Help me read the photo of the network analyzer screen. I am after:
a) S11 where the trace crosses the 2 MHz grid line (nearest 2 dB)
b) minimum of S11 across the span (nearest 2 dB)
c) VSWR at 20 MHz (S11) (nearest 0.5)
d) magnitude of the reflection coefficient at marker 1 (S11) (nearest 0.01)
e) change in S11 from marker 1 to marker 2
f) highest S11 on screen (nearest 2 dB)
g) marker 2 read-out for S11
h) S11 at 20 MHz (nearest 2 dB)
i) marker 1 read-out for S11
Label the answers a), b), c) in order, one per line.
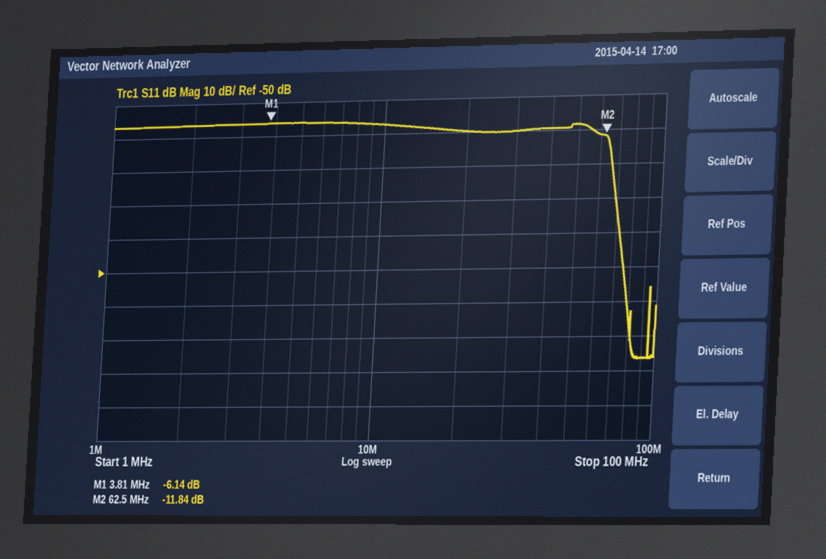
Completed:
a) -6 dB
b) -76 dB
c) 2.0
d) 0.49
e) -5.70 dB
f) -6 dB
g) -11.84 dB
h) -10 dB
i) -6.14 dB
